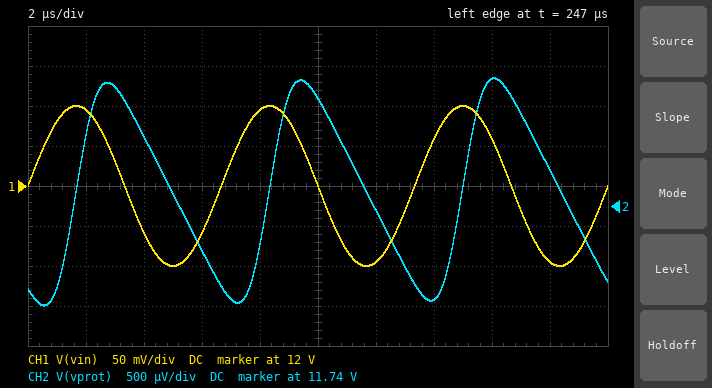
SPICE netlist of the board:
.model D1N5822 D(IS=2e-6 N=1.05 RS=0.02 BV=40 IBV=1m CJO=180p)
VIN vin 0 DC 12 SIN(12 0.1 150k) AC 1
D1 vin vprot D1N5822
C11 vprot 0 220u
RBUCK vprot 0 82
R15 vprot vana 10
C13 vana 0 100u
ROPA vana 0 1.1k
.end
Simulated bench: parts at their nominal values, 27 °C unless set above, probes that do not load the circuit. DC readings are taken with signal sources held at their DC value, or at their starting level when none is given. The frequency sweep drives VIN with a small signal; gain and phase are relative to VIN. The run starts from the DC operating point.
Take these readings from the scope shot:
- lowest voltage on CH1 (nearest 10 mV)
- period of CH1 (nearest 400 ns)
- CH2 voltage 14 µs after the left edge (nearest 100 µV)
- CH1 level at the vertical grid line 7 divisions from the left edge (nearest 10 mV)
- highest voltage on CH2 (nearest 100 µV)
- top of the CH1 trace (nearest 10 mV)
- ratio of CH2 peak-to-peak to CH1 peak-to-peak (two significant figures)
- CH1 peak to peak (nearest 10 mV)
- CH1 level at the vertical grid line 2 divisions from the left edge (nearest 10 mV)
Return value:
11.90 V
6.8 µs
11.7413 V
12.06 V
11.7441 V
12.10 V
0.014
200 mV
11.94 V
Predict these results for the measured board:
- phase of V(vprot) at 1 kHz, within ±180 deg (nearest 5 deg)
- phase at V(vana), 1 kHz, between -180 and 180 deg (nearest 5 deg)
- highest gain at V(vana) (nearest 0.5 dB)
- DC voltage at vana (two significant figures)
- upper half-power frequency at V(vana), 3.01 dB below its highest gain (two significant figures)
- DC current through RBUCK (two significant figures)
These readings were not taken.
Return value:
-15 deg
-95 deg
0 dB
12 V
160 Hz
140 mA
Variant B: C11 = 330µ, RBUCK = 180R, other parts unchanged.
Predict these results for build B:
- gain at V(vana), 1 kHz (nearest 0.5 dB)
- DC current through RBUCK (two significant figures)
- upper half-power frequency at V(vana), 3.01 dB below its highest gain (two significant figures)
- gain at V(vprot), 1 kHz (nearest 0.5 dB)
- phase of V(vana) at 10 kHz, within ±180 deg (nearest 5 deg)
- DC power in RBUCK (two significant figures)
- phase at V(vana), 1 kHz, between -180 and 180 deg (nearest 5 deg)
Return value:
-18.5 dB
65 mA
150 Hz
-2.5 dB
-170 deg
760 mW
-120 deg
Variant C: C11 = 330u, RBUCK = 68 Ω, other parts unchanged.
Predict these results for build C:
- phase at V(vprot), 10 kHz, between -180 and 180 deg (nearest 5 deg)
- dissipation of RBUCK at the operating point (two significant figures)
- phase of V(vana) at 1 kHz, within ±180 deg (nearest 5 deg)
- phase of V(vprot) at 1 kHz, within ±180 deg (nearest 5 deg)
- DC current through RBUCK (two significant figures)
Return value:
-75 deg
2.0 W
-100 deg
-20 deg
170 mA
